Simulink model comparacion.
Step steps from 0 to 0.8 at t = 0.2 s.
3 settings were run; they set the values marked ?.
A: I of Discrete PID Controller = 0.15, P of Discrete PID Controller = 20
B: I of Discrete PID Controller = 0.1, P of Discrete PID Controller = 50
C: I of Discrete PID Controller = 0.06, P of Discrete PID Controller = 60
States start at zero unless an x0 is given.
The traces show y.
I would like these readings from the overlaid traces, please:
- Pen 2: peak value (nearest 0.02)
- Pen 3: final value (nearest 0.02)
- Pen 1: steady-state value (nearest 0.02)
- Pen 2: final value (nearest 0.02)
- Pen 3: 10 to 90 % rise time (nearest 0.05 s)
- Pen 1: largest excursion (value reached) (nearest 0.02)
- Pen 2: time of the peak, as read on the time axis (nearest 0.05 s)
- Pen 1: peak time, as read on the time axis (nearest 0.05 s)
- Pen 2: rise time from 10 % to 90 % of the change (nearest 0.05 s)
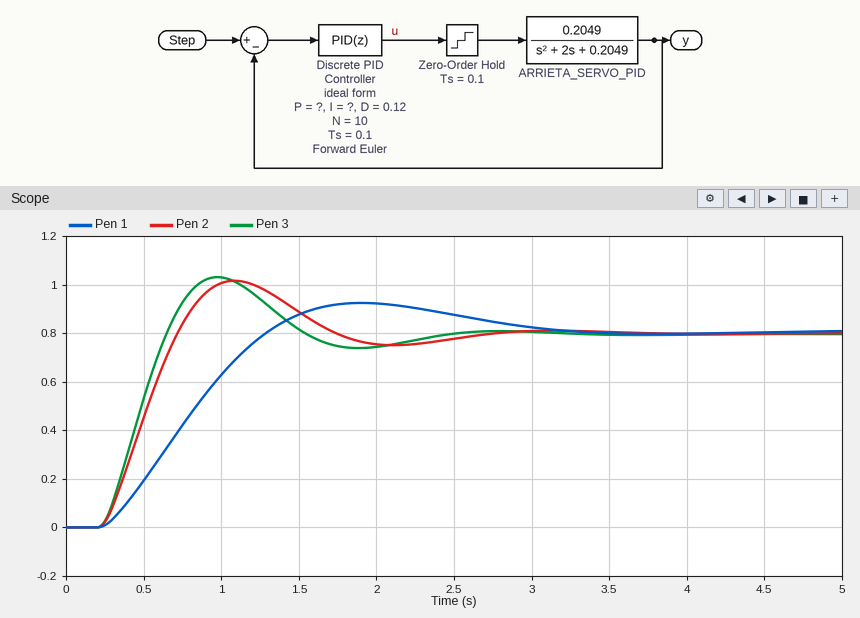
1.02
0.80
0.80
0.80
0.30 s
0.92
1.10 s
1.90 s
0.35 s
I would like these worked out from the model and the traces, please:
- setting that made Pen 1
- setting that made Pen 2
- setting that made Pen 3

A
B
C
